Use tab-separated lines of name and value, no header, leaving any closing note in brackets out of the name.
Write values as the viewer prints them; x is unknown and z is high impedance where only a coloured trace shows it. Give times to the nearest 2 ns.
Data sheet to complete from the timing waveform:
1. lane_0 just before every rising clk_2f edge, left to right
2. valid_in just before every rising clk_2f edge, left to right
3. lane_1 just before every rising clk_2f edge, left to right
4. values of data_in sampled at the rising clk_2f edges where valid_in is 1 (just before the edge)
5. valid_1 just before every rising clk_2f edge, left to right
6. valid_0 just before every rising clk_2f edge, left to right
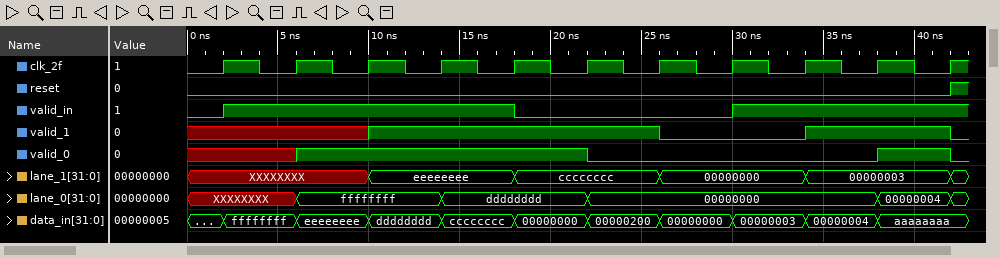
lane_0 just before every rising clk_2f edge, left to right	XXXXXXXX, XXXXXXXX, ffffffff, ffffffff, dddddddd, dddddddd, 00000000, 00000000, 00000000, 00000000, 00000004
valid_in just before every rising clk_2f edge, left to right	0 1 1 1 1 0 0 0 1 1 1
lane_1 just before every rising clk_2f edge, left to right	XXXXXXXX, XXXXXXXX, XXXXXXXX, eeeeeeee, eeeeeeee, cccccccc, cccccccc, 00000000, 00000000, 00000003, 00000003
values of data_in sampled at the rising clk_2f edges where valid_in is 1	ffffffff, eeeeeeee, dddddddd, cccccccc, 00000003, 00000004, aaaaaaaa
valid_1 just before every rising clk_2f edge, left to right	x x x 1 1 1 1 0 0 1 1
valid_0 just before every rising clk_2f edge, left to right	x x 1 1 1 1 0 0 0 0 1
